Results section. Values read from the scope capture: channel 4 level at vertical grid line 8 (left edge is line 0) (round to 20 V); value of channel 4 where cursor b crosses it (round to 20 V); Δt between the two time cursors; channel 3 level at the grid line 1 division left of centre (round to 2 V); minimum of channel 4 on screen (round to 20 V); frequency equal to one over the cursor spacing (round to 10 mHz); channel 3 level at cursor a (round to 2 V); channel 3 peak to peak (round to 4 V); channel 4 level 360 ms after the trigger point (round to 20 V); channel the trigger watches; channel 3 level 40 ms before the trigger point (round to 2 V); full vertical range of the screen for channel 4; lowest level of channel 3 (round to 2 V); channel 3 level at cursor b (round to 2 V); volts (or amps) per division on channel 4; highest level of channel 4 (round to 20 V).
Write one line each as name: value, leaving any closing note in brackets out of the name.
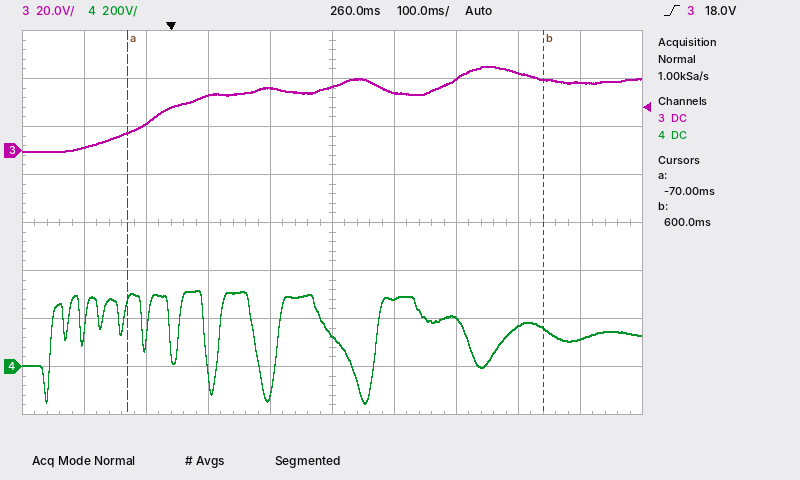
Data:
channel 4 level at vertical grid line 8 (left edge is line 0): 160 V
value of channel 4 where cursor b crosses it: 160 V
Δt between the two time cursors: 670 ms
channel 3 level at the grid line 1 division left of centre: 26 V
minimum of channel 4 on screen: -160 V
frequency equal to one over the cursor spacing: 1.49 Hz
channel 3 level at cursor a: 8 V
channel 3 peak to peak: 36 V
channel 4 level 360 ms after the trigger point: 280 V
channel the trigger watches: channel 3
channel 3 level 40 ms before the trigger point: 12 V
full vertical range of the screen for channel 4: 1.6 kV
lowest level of channel 3: 0 V
channel 3 level at cursor b: 30 V
volts (or amps) per division on channel 4: 200 V
highest level of channel 4: 320 V
